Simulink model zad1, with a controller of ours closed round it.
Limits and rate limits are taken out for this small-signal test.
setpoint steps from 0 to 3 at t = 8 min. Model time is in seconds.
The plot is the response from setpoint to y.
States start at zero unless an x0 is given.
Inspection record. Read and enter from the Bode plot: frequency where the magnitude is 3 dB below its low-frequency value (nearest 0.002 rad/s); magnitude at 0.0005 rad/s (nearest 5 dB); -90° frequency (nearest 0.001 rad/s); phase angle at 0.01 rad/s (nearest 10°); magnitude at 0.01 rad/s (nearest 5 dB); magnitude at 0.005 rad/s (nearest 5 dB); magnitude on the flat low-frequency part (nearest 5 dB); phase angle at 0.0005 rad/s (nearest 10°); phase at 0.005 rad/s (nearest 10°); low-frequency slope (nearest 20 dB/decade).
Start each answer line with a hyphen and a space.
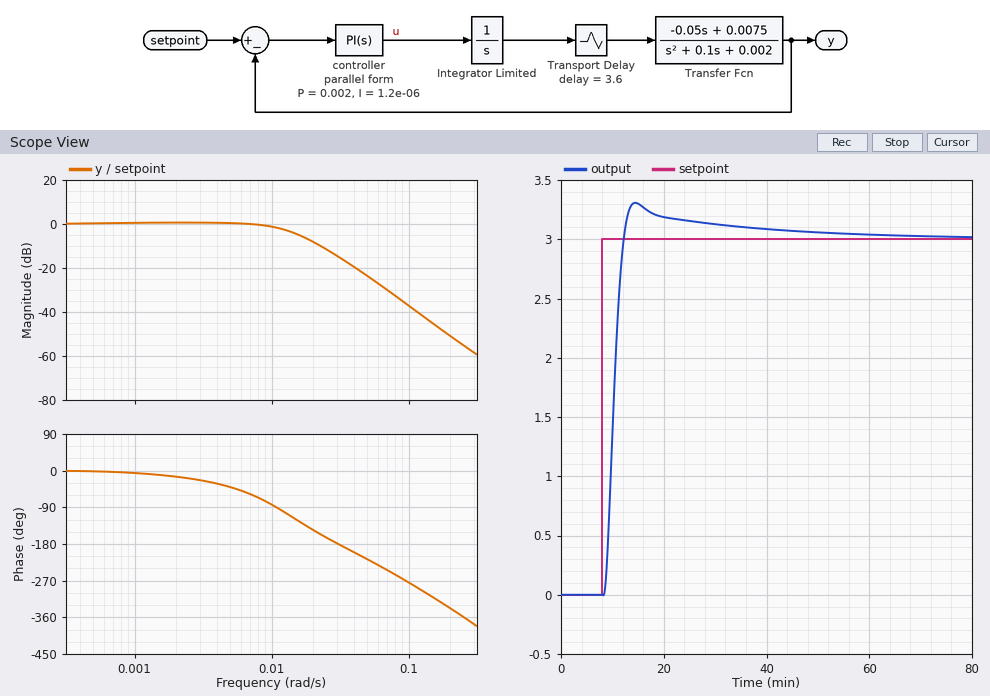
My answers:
- 0.012 rad/s
- 0 dB
- 0.011 rad/s
- -80°
- 0 dB
- 0 dB
- 0 dB
- 0°
- -40°
- 0 dB/decade
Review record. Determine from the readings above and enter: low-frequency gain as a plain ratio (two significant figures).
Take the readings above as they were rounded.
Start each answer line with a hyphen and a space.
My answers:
- 1.0
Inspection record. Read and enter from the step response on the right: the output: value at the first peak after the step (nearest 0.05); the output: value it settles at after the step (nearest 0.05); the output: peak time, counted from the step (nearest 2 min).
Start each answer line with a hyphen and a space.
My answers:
- 3.30
- 3.00
- 6 min
